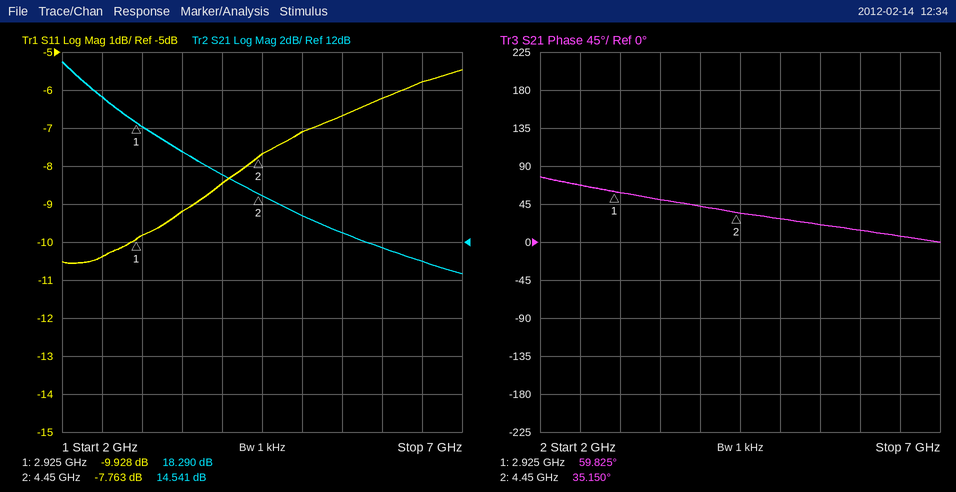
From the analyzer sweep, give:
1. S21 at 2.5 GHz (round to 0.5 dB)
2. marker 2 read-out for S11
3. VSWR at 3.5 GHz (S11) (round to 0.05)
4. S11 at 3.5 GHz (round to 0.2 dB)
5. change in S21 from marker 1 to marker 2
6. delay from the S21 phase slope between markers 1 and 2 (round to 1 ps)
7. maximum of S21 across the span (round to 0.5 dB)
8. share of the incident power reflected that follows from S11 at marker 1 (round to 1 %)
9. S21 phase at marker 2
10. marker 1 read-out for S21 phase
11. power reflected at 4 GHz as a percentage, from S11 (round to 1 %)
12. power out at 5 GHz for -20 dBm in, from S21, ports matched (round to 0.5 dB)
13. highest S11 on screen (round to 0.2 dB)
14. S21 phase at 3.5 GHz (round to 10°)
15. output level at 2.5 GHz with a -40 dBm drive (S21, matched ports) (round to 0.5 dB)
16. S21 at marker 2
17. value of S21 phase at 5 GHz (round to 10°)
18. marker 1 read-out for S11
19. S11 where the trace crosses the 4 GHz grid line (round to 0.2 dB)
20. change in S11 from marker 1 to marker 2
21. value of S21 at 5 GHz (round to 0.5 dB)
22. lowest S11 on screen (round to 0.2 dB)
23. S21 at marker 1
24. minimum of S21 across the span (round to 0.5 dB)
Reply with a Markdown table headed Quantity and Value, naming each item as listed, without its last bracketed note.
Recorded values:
| Quantity | Value |
|---|---|
| S21 at 2.5 GHz | 19.5 dB |
| marker 2 read-out for S11 | -7.763 dB |
| VSWR at 3.5 GHz (S11) | 2.05 |
| S11 at 3.5 GHz | -9.2 dB |
| change in S21 from marker 1 to marker 2 | -3.749 dB |
| delay from the S21 phase slope between markers 1 and 2 | 45 ps |
| maximum of S21 across the span | 21.5 dB |
| share of the incident power reflected that follows from S11 at marker 1 | 10 % |
| S21 phase at marker 2 | 35.150° |
| marker 1 read-out for S21 phase | 59.825° |
| power reflected at 4 GHz as a percentage, from S11 | 14 % |
| power out at 5 GHz for -20 dBm in, from S21, ports matched | -6.5 dBm |
| highest S11 on screen | -5.4 dB |
| S21 phase at 3.5 GHz | 50° |
| output level at 2.5 GHz with a -40 dBm drive (S21, matched ports) | -20.5 dBm |
| S21 at marker 2 | 14.541 dB |
| value of S21 phase at 5 GHz | 30° |
| marker 1 read-out for S11 | -9.928 dB |
| S11 where the trace crosses the 4 GHz grid line | -8.4 dB |
| change in S11 from marker 1 to marker 2 | 2.165 dB |
| value of S21 at 5 GHz | 13.5 dB |
| lowest S11 on screen | -10.6 dB |
| S21 at marker 1 | 18.290 dB |
| minimum of S21 across the span | 10.5 dB |
